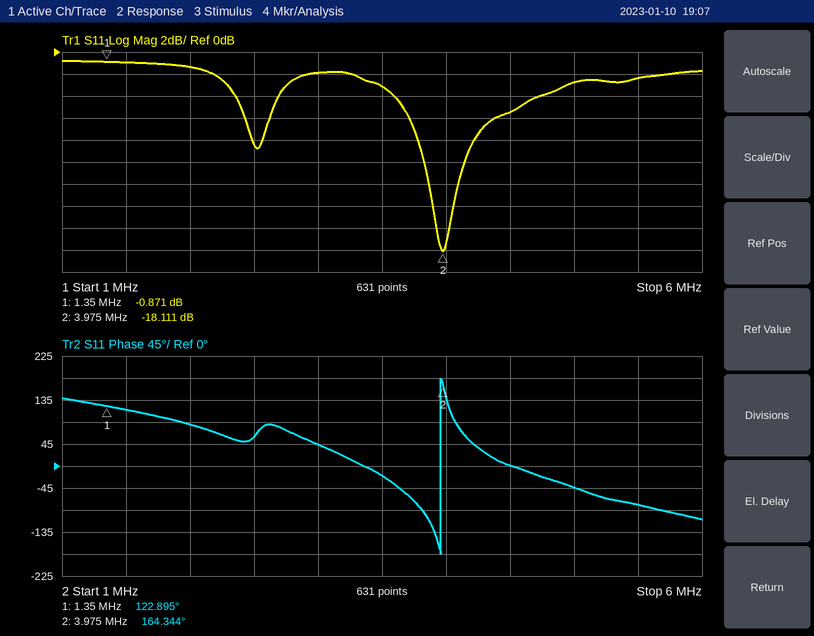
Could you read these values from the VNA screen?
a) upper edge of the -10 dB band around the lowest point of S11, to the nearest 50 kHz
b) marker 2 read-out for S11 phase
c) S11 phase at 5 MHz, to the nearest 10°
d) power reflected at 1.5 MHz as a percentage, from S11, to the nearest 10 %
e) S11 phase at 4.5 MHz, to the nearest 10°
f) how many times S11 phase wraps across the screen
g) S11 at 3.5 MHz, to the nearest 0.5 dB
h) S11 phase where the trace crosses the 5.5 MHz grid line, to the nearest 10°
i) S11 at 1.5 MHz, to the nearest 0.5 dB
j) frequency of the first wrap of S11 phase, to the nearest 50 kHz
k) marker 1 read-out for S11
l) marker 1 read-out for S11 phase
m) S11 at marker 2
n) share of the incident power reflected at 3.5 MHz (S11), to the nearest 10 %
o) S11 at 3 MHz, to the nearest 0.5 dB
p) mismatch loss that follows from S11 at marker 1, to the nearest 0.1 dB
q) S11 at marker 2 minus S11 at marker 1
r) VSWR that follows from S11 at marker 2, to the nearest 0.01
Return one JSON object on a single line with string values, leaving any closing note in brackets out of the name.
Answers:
{"upper edge of the -10 dB band around the lowest point of S11, to the nearest 50 kHz": "4.15 MHz", "marker 2 read-out for S11 phase": "164.344°", "S11 phase at 5 MHz, to the nearest 10°": "-40°", "power reflected at 1.5 MHz as a percentage, from S11, to the nearest 10 %": "80 %", "S11 phase at 4.5 MHz, to the nearest 10°": "0°", "how many times S11 phase wraps across the screen": "1", "S11 at 3.5 MHz, to the nearest 0.5 dB": "-3.0 dB", "S11 phase where the trace crosses the 5.5 MHz grid line, to the nearest 10°": "-80°", "S11 at 1.5 MHz, to the nearest 0.5 dB": "-1.0 dB", "frequency of the first wrap of S11 phase, to the nearest 50 kHz": "3.95 MHz", "marker 1 read-out for S11": "-0.871 dB", "marker 1 read-out for S11 phase": "122.895°", "S11 at marker 2": "-18.111 dB", "share of the incident power reflected at 3.5 MHz (S11), to the nearest 10 %": "50 %", "S11 at 3 MHz, to the nearest 0.5 dB": "-2.0 dB", "mismatch loss that follows from S11 at marker 1, to the nearest 0.1 dB": "7.4 dB", "S11 at marker 2 minus S11 at marker 1": "-17.240 dB", "VSWR that follows from S11 at marker 2, to the nearest 0.01": "1.28"}
